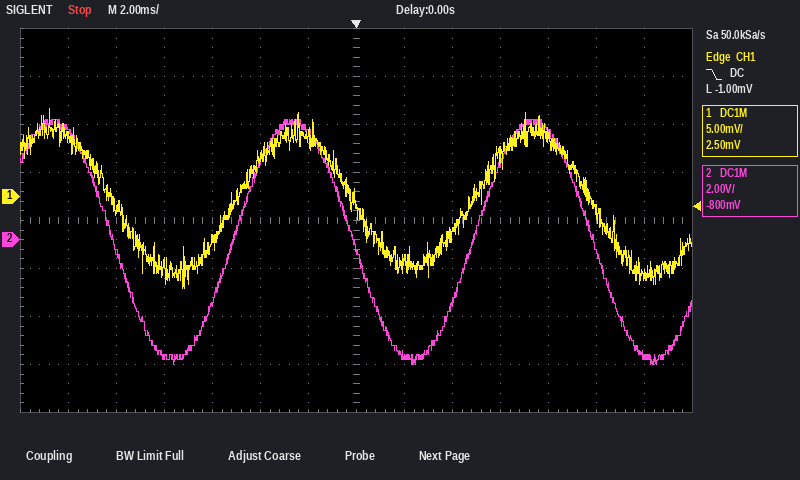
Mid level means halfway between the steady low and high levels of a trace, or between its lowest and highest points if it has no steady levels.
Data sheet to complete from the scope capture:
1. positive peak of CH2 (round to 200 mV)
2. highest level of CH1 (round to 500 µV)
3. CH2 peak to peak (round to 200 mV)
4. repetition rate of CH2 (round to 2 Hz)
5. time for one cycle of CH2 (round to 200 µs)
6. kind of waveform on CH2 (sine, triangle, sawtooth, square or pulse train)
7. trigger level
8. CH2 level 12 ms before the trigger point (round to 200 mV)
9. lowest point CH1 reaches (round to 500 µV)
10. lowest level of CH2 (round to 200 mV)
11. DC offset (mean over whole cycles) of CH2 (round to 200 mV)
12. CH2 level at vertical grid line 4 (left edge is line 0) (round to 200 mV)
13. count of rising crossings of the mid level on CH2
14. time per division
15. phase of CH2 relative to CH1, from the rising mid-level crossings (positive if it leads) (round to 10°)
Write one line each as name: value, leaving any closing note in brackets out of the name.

positive peak of CH2: 5.0 V
highest level of CH1: 9.0 mV
CH2 peak to peak: 10.2 V
repetition rate of CH2: 100 Hz
time for one cycle of CH2: 10.0 ms
kind of waveform on CH2: sine
trigger level: -1.00 mV
CH2 level 12 ms before the trigger point: 4.6 V
lowest point CH1 reaches: -9.5 mV
lowest level of CH2: -5.2 V
DC offset (mean over whole cycles) of CH2: 0.0 V
CH2 level at vertical grid line 4 (left edge is line 0): -2.6 V
count of rising crossings of the mid level on CH2: 2
time per division: 2 ms
phase of CH2 relative to CH1, from the rising mid-level crossings (positive if it leads): 0°
